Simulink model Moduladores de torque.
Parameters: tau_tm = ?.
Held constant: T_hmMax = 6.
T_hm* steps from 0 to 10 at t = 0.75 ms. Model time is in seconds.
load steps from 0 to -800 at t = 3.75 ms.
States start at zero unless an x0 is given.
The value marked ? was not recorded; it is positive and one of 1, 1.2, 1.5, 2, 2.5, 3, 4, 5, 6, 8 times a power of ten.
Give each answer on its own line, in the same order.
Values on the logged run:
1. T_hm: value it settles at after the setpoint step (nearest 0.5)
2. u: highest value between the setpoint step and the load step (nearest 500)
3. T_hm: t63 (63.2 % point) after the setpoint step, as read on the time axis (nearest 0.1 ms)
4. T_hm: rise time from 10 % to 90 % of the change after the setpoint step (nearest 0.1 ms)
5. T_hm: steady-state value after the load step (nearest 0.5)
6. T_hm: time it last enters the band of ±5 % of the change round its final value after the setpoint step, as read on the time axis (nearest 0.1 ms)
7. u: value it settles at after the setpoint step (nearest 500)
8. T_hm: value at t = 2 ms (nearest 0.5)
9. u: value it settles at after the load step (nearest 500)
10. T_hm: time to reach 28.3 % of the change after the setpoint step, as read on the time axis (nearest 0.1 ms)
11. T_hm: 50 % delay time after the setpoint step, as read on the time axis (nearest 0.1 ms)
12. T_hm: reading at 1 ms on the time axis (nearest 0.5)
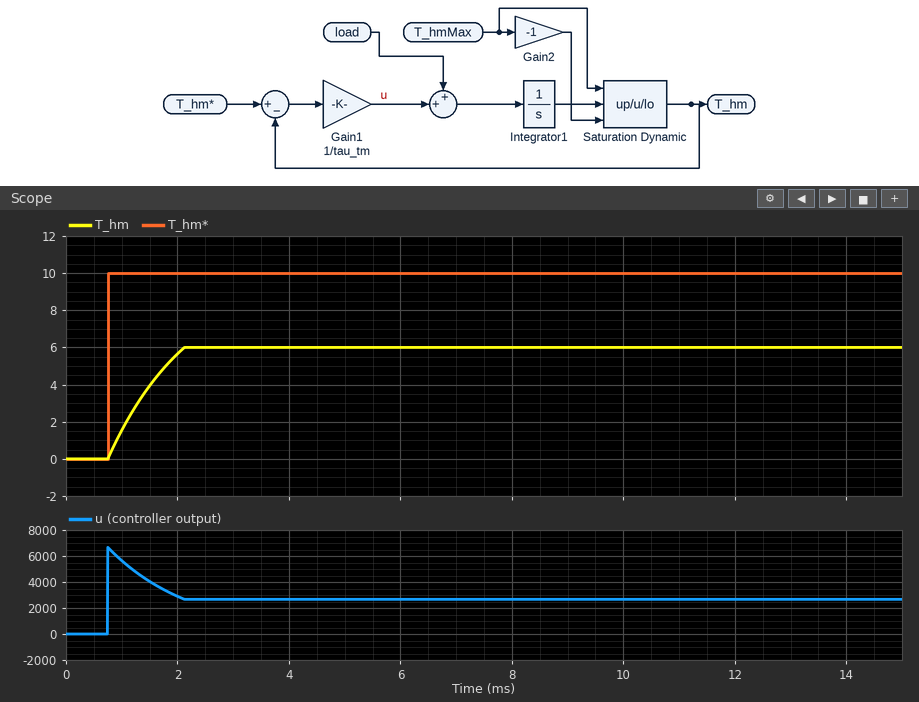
6.0
6500
1.5 ms
1.1 ms
6.0
2.0 ms
2500
5.5
2500
1.0 ms
1.3 ms
1.5
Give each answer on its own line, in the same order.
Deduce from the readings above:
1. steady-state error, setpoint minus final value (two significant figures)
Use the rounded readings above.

4.0
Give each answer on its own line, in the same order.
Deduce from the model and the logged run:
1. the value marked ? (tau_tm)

0.0015
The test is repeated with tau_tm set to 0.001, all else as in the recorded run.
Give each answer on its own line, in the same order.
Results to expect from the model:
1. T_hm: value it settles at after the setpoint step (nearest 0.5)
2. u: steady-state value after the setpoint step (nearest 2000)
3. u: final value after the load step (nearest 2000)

6.0
4000
4000
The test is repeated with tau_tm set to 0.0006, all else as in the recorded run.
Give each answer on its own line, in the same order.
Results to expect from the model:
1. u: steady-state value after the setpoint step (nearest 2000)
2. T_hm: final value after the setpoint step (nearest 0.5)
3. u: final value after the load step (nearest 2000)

6000
6.0
6000
